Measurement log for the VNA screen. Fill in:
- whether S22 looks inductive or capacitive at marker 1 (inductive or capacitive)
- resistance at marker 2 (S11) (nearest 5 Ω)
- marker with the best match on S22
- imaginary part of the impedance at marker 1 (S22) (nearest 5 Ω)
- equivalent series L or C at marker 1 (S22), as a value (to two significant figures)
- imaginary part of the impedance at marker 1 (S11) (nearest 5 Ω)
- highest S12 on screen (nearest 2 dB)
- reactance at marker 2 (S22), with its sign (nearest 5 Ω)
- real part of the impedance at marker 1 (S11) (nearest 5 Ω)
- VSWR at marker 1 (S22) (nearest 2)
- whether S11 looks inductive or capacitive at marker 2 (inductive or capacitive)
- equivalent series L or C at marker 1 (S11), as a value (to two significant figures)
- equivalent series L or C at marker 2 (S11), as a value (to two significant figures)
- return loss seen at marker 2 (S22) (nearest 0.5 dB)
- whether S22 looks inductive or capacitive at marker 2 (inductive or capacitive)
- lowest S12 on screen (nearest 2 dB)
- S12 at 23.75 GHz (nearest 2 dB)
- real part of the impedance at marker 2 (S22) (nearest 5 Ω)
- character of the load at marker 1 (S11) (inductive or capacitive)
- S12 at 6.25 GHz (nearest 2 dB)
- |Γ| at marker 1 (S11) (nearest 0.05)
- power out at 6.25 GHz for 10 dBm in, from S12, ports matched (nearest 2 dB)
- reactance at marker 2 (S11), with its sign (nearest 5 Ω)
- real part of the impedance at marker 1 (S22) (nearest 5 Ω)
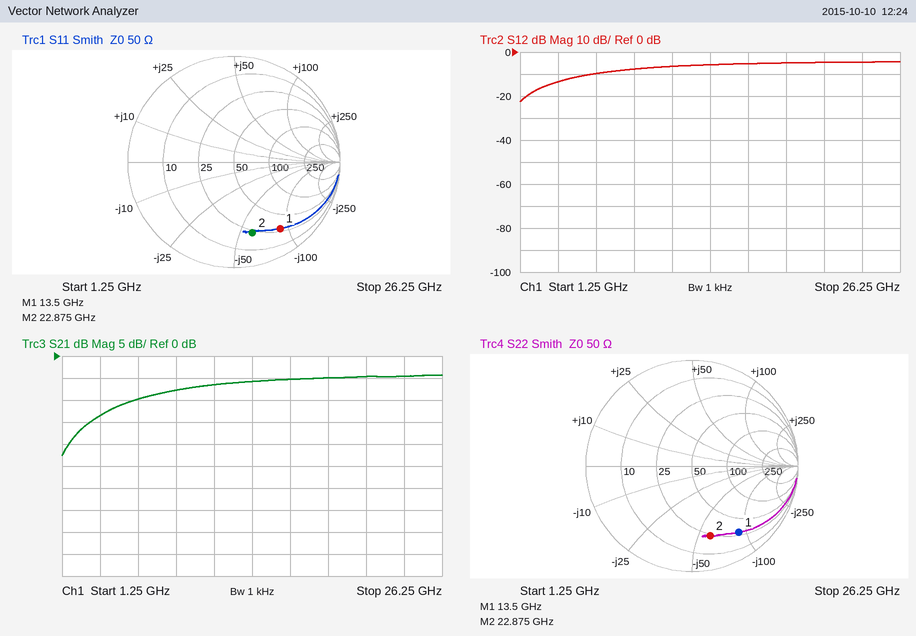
capacitive
25 Ω
marker 2
-90 Ω
130 fF
-90 Ω
-4 dB
-60 Ω
30 Ω
8
capacitive
130 fF
120 fF
3.5 dB
capacitive
-22 dB
-4 dB
25 Ω
capacitive
-10 dB
0.75
0 dBm
-60 Ω
30 Ω
